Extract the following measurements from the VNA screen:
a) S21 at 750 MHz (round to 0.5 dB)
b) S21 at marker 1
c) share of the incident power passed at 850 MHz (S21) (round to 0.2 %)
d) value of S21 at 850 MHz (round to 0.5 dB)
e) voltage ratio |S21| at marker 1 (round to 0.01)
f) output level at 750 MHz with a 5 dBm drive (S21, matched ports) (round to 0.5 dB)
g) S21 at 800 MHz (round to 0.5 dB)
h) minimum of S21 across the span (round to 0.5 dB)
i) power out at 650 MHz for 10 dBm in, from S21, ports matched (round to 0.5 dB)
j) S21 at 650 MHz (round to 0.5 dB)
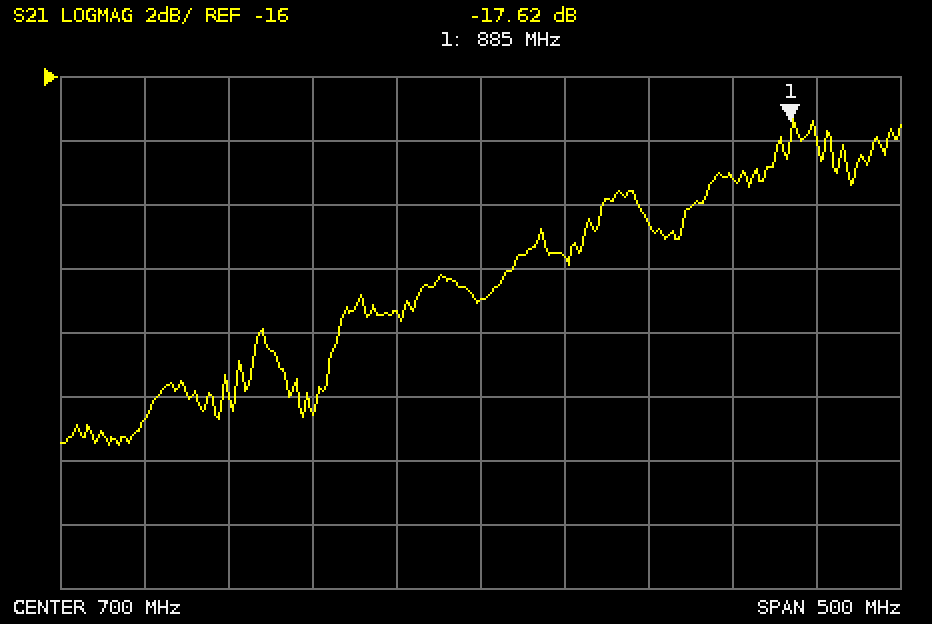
-21.5 dB
-17.62 dB
1.2 %
-19.0 dB
0.13
-16.5 dBm
-20.5 dB
-27.5 dB
-13.5 dBm
-23.5 dB
